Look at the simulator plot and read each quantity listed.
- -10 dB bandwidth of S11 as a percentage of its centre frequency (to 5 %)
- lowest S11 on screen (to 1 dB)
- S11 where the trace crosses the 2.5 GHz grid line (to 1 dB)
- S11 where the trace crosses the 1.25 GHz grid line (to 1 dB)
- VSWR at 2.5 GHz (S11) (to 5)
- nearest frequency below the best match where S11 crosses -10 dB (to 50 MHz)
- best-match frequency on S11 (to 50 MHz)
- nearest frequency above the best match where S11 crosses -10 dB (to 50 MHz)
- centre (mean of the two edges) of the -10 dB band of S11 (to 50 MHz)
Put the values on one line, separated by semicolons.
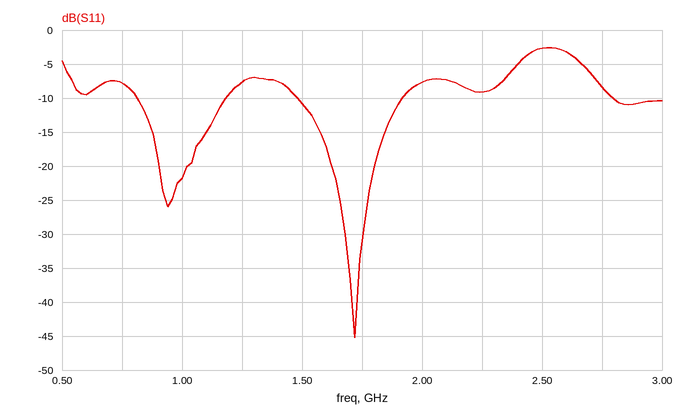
25 %; -45 dB; -3 dB; -8 dB; 5; 1.50 GHz; 1.70 GHz; 1.90 GHz; 1.70 GHz
